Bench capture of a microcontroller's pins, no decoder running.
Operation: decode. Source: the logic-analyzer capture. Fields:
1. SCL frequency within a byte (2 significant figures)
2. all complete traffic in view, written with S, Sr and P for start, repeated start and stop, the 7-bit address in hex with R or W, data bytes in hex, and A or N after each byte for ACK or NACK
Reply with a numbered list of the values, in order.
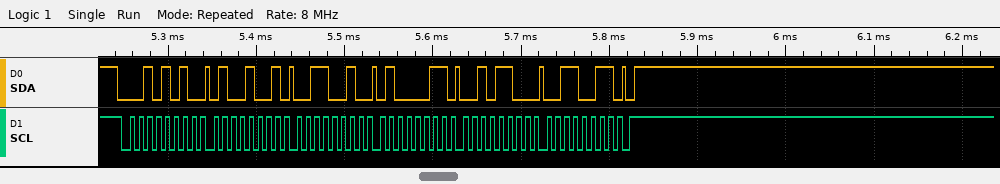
1. 100 kHz
2. S 15W A 49 A 32 A 43 A 2C A 33 A P
